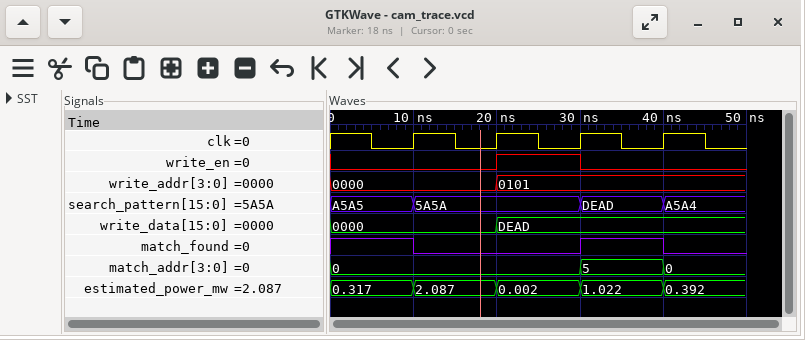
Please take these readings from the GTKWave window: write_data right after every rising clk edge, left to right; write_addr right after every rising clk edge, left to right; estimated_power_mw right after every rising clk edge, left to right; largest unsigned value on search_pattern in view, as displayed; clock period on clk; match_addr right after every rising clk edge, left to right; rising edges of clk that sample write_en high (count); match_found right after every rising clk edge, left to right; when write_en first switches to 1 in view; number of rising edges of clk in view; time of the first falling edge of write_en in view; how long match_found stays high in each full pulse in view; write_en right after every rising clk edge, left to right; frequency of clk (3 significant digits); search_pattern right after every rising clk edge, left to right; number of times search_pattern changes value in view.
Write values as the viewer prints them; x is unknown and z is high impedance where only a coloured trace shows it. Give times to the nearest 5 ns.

0000, DEAD, DEAD, DEAD
0000, 0101, 0101, 0101
2.087, 0.002, 1.022, 0.392
DEAD
10 ns
0, 0, 5, 0
1
0 0 1 0
20 ns
4
30 ns
10 ns
0 1 0 0
100 MHz
5A5A, 5A5A, DEAD, A5A4
3
